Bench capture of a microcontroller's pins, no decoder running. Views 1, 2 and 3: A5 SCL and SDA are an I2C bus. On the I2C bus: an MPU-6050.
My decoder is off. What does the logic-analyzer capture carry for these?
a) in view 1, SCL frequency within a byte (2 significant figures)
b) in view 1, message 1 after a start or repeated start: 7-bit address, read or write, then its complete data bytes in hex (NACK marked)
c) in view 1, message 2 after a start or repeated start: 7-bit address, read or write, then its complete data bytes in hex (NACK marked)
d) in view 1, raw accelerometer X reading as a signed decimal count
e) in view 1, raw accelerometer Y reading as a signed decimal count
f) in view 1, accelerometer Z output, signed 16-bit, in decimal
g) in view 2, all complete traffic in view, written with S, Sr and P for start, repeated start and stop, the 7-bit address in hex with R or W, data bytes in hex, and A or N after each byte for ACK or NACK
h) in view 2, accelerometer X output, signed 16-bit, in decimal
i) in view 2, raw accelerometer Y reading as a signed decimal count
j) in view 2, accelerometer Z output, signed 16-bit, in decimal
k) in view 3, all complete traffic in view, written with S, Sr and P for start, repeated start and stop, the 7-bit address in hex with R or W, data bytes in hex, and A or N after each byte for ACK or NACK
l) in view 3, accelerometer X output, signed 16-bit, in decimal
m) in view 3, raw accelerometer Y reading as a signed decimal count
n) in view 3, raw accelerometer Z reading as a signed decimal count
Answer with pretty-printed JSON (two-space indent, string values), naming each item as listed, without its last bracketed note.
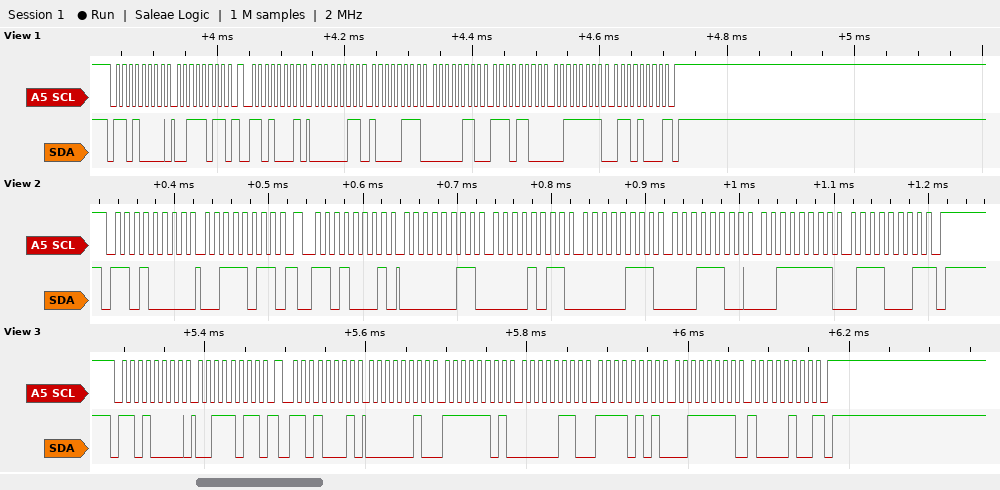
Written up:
{
  "in view 1, SCL frequency within a byte": "100 kHz",
  "in view 1, message 1 after a start or repeated start: 7-bit address, read or write, then its complete data bytes in hex": "0x68 write: 3B",
  "in view 1, message 2 after a start or repeated start: 7-bit address, read or write, then its complete data bytes in hex": "0x68 read: 03 87 06 EC 3F 68 NACK",
  "in view 1, raw accelerometer X reading as a signed decimal count": "903",
  "in view 1, raw accelerometer Y reading as a signed decimal count": "1772",
  "in view 1, accelerometer Z output, signed 16-bit, in decimal": "16232",
  "in view 2, all complete traffic in view, written with S, Sr and P for start, repeated start and stop, the 7-bit address in hex with R or W, data bytes in hex, and A or N after each byte for ACK or NACK": "S 68W A 3B A Sr 68R A 03 A 0B A 07 A 1C A 3F A 71 N P",
  "in view 2, accelerometer X output, signed 16-bit, in decimal": "779",
  "in view 2, raw accelerometer Y reading as a signed decimal count": "1820",
  "in view 2, accelerometer Z output, signed 16-bit, in decimal": "16241",
  "in view 3, all complete traffic in view, written with S, Sr and P for start, repeated start and stop, the 7-bit address in hex with R or W, data bytes in hex, and A or N after each byte for ACK or NACK": "S 68W A 3B A Sr 68R A 02 A FD A 06 A F5 A 3F A 84 N P",
  "in view 3, accelerometer X output, signed 16-bit, in decimal": "765",
  "in view 3, raw accelerometer Y reading as a signed decimal count": "1781",
  "in view 3, raw accelerometer Z reading as a signed decimal count": "16260"
}
